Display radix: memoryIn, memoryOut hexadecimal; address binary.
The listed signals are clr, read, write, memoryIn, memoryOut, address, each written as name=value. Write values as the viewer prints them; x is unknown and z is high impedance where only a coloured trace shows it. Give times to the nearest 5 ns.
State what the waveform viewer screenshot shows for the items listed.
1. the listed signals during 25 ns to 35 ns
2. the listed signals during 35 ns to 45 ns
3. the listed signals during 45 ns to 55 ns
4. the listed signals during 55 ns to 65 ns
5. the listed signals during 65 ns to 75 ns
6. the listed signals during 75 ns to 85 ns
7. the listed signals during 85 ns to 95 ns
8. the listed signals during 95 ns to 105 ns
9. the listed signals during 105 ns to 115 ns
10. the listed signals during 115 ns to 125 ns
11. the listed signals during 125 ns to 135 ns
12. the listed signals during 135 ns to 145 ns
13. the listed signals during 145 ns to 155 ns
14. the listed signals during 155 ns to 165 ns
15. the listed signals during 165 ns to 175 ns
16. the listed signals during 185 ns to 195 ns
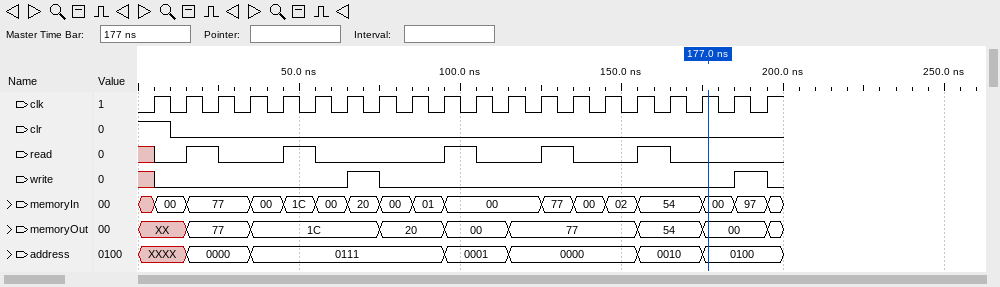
clr=0, read=0, write=0, memoryIn=77, memoryOut=77, address=0000
clr=0, read=0, write=0, memoryIn=00, memoryOut=1C, address=0111
clr=0, read=1, write=0, memoryIn=1C, memoryOut=1C, address=0111
clr=0, read=0, write=0, memoryIn=00, memoryOut=1C, address=0111
clr=0, read=0, write=1, memoryIn=20, memoryOut=1C, address=0111
clr=0, read=0, write=0, memoryIn=00, memoryOut=20, address=0111
clr=0, read=0, write=0, memoryIn=01, memoryOut=20, address=0111
clr=0, read=1, write=0, memoryIn=00, memoryOut=00, address=0001
clr=0, read=0, write=0, memoryIn=00, memoryOut=00, address=0001
clr=0, read=0, write=0, memoryIn=00, memoryOut=77, address=0000
clr=0, read=1, write=0, memoryIn=77, memoryOut=77, address=0000
clr=0, read=0, write=0, memoryIn=00, memoryOut=77, address=0000
clr=0, read=0, write=0, memoryIn=02, memoryOut=77, address=0000
clr=0, read=1, write=0, memoryIn=54, memoryOut=54, address=0010
clr=0, read=0, write=0, memoryIn=54, memoryOut=54, address=0010
clr=0, read=0, write=1, memoryIn=97, memoryOut=00, address=0100
